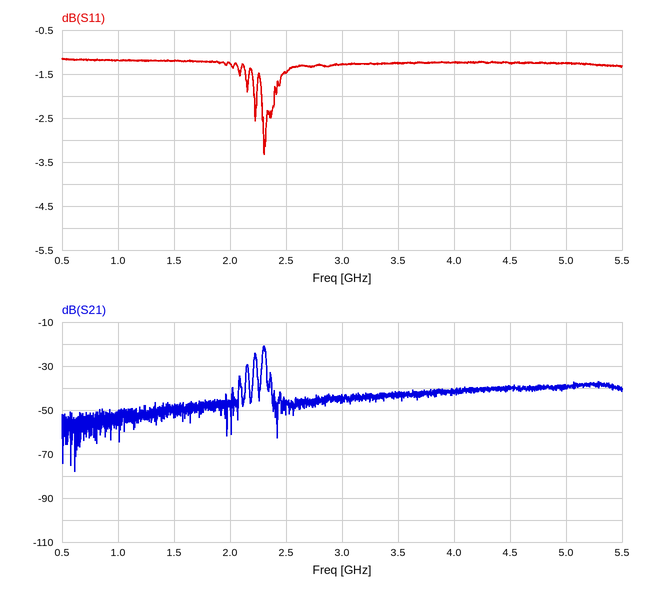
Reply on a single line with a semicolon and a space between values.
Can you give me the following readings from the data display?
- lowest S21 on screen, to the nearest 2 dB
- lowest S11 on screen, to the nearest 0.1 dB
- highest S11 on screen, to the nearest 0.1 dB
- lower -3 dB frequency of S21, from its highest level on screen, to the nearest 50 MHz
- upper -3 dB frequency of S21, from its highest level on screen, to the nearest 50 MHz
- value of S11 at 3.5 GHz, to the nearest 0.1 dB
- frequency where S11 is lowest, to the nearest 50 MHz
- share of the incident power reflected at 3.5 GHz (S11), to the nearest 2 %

-78 dB; -3.3 dB; -1.1 dB; 2.30 GHz; 2.30 GHz; -1.2 dB; 2.30 GHz; 76 %
